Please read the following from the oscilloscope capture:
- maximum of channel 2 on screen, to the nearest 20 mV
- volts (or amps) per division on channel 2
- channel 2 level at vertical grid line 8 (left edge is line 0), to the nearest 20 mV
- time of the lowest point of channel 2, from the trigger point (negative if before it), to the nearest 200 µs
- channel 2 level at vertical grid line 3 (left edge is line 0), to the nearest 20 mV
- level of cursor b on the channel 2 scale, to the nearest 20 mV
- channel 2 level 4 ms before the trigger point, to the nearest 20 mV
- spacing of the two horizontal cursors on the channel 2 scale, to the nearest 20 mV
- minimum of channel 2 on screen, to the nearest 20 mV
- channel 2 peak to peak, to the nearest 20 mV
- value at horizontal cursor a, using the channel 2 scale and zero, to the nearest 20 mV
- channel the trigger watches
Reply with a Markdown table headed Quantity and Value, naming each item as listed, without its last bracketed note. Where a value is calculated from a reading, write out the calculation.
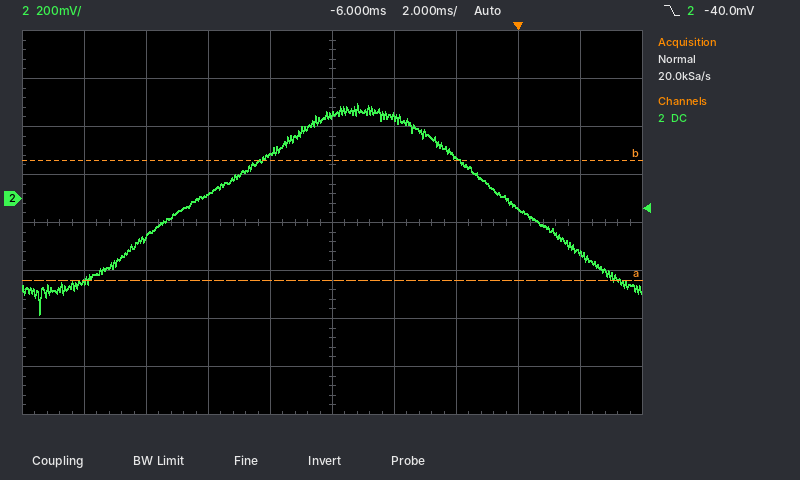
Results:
| Quantity | Value |
|---|---|
| maximum of channel 2 on screen, to the nearest 20 mV | 400 mV |
| volts (or amps) per division on channel 2 | 200 mV |
| channel 2 level at vertical grid line 8 (left edge is line 0), to the nearest 20 mV | -40 mV |
| time of the lowest point of channel 2, from the trigger point (negative if before it), to the nearest 200 µs | -15.4 ms |
| channel 2 level at vertical grid line 3 (left edge is line 0), to the nearest 20 mV | 20 mV |
| level of cursor b on the channel 2 scale, to the nearest 20 mV | 160 mV |
| channel 2 level 4 ms before the trigger point, to the nearest 20 mV | 340 mV |
| spacing of the two horizontal cursors on the channel 2 scale, to the nearest 20 mV | 500 mV |
| minimum of channel 2 on screen, to the nearest 20 mV | -480 mV |
| channel 2 peak to peak, to the nearest 20 mV | 400 mV − (-480 mV) = 880 mV |
| value at horizontal cursor a, using the channel 2 scale and zero, to the nearest 20 mV | -340 mV |
| channel the trigger watches | channel 2 |
